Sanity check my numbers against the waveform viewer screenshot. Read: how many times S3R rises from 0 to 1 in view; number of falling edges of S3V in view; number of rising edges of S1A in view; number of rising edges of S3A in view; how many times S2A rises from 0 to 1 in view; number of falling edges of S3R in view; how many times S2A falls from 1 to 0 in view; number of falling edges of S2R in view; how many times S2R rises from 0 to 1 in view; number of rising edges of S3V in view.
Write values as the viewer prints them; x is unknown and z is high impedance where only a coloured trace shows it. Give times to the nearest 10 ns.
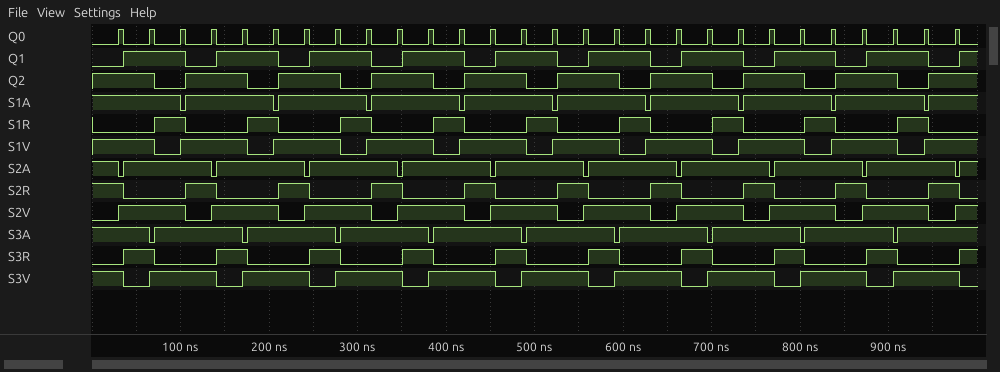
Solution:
10
10
9
9
10
9
10
10
9
9
